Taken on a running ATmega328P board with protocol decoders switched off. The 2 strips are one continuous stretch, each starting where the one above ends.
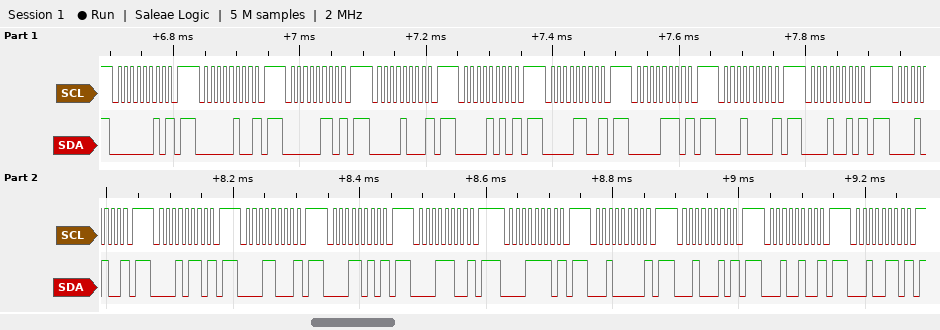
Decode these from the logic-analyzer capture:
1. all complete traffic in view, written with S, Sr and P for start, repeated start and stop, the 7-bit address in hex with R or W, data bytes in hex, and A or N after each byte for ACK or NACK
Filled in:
S 01W N P S 02W N P S 03W N P S 04W N P S 05W N P S 06W N P S 07W N P S 08W N P S 09W N P S 0AW N P S 0BW N P S 0CW N P S 0DW N P S 0EW N P S 0FW N P S 10W N P S 11W N P S 12W N P S 13W N P
